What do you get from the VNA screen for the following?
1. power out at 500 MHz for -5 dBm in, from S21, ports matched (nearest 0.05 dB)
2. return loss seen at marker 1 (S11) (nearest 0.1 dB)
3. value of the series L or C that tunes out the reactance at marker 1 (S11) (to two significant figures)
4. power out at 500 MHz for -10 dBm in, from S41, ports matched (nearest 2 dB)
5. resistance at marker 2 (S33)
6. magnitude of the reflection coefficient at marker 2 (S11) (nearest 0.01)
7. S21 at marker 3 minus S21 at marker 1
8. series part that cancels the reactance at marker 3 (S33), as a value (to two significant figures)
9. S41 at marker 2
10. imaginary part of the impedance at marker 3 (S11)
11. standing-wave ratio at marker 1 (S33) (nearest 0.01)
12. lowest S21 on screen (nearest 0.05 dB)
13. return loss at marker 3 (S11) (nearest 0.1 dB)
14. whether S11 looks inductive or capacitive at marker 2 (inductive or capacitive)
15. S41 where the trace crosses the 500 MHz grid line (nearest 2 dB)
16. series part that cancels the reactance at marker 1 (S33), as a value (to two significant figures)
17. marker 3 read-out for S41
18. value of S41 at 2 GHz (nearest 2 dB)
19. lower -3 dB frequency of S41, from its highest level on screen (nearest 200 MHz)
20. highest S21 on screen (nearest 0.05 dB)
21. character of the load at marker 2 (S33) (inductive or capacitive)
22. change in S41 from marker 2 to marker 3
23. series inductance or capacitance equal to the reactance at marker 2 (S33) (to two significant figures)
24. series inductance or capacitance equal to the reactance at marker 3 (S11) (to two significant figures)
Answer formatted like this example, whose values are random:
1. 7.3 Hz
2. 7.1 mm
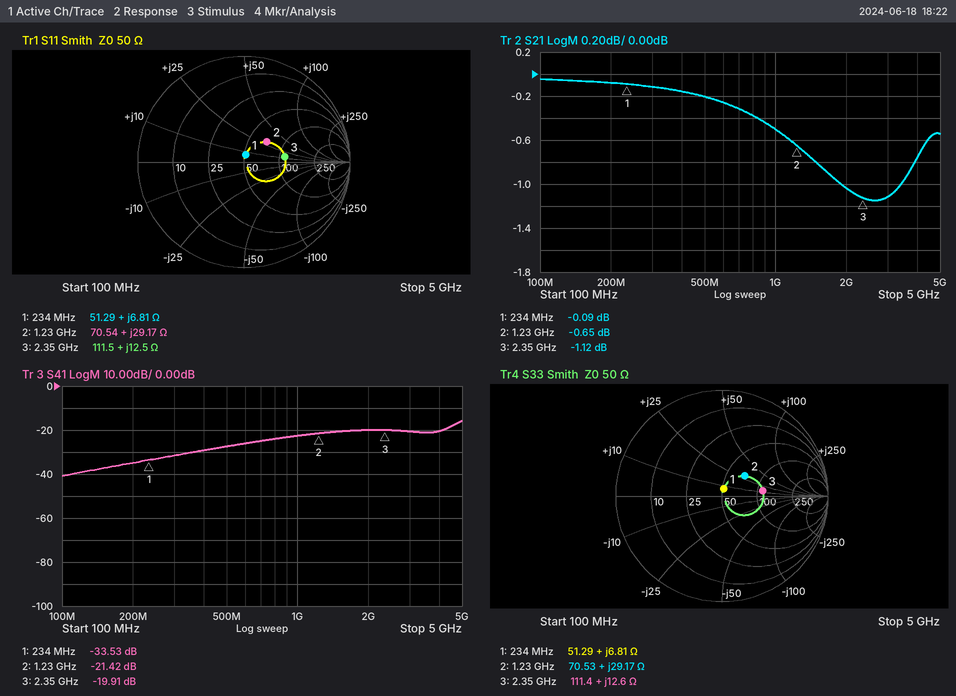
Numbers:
1. -5.20 dBm
2. 23.3 dB
3. 100 pF
4. -38 dBm
5. 70.53 Ω
6. 0.29
7. -1.03 dB
8. 5.4 pF
9. -21.42 dB
10. +12.5 Ω
11. 1.15
12. -1.15 dB
13. 8.2 dB
14. inductive
15. -28 dB
16. 100 pF
17. -19.91 dB
18. -20 dB
19. 4.4 GHz
20. -0.05 dB
21. inductive
22. 1.51 dB
23. 3.8 nH
24. 850 pH
